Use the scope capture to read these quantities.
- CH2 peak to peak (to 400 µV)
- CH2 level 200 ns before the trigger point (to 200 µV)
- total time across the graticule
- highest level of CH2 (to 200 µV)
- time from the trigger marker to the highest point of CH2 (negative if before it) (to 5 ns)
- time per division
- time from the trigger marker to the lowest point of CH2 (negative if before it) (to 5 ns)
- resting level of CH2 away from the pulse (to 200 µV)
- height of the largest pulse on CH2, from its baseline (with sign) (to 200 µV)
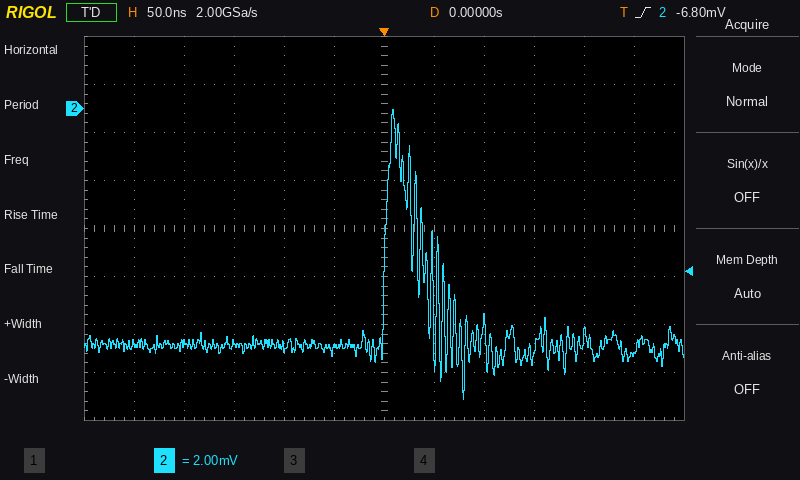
12.0 mV
-9.8 mV
600 ns
0.0 mV
+10 ns
50 ns
+80 ns
-9.8 mV
+9.8 mV
